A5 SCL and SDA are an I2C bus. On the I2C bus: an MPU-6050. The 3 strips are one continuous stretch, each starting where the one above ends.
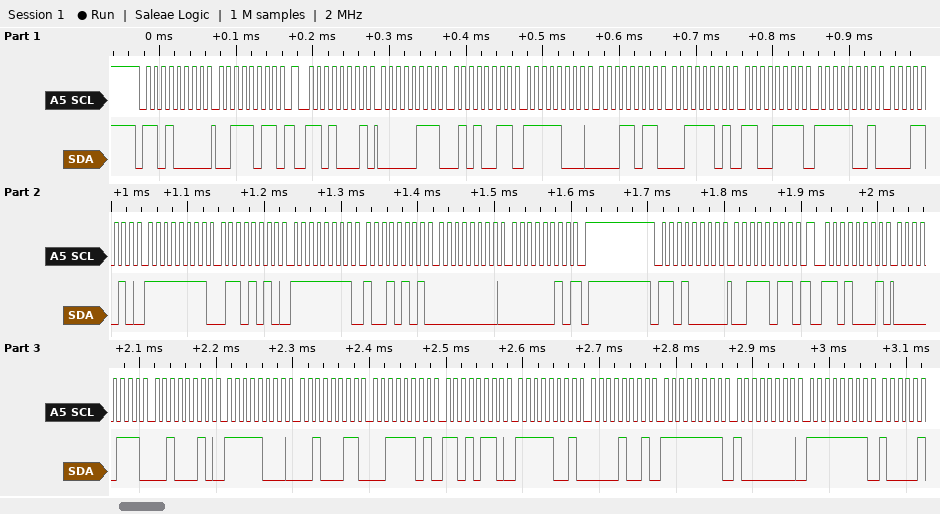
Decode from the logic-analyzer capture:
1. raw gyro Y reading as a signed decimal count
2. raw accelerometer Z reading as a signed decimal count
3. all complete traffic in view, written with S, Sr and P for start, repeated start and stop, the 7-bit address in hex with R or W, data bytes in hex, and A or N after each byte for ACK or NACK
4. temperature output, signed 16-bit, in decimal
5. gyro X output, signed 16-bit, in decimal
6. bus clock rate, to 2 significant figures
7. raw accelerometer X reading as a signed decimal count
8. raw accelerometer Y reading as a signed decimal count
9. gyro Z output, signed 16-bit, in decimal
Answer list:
-107
15823
S 68W A 3B A Sr 68R A 07 A 53 A F8 A 1B A 3D A CF A F9 A 1A A FF A 6A A FF A 95 A 00 A 02 N P S 68W A 3B A Sr 68R A 07 A 22 A F8 A 23 A 3D A D6 A F9 A 09 A FF A 80 A FF A
-1766
-150
100 kHz
1875
-2021
2
